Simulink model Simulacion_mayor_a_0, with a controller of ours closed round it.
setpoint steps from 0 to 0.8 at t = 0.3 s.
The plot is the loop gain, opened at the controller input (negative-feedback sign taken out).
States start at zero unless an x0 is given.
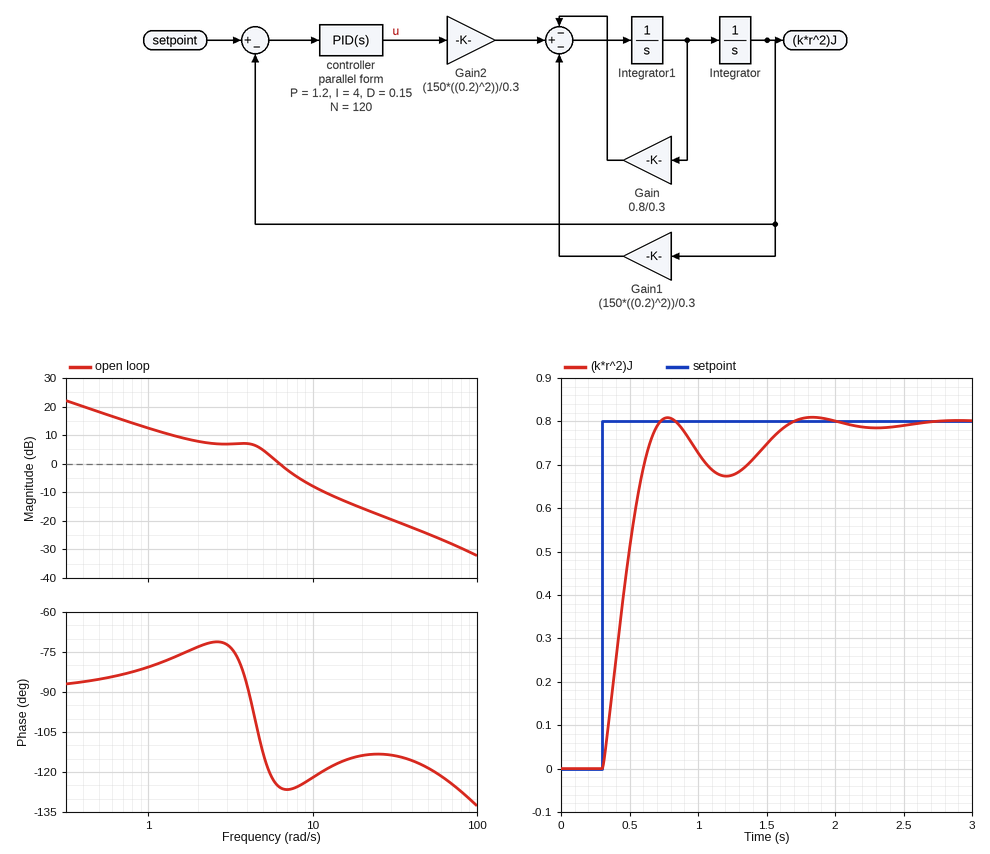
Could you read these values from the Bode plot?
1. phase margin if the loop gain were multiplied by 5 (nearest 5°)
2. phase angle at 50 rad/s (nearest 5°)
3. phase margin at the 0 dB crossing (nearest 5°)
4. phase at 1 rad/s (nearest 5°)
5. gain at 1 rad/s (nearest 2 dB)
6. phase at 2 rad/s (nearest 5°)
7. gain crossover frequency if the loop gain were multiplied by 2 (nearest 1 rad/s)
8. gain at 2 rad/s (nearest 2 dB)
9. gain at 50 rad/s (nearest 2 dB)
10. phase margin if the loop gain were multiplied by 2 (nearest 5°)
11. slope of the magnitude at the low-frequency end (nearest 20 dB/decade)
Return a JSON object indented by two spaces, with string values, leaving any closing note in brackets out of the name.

{
  "phase margin if the loop gain were multiplied by 5": "65°",
  "phase angle at 50 rad/s": "-120°",
  "phase margin at the 0 dB crossing": "55°",
  "phase at 1 rad/s": "-80°",
  "gain at 1 rad/s": "12 dB",
  "phase at 2 rad/s": "-75°",
  "gain crossover frequency if the loop gain were multiplied by 2": "9 rad/s",
  "gain at 2 rad/s": "8 dB",
  "gain at 50 rad/s": "-24 dB",
  "phase margin if the loop gain were multiplied by 2": "55°",
  "slope of the magnitude at the low-frequency end": "-20 dB/decade"
}
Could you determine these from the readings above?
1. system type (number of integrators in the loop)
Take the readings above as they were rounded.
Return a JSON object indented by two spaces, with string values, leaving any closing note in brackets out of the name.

{
  "system type": "1"
}
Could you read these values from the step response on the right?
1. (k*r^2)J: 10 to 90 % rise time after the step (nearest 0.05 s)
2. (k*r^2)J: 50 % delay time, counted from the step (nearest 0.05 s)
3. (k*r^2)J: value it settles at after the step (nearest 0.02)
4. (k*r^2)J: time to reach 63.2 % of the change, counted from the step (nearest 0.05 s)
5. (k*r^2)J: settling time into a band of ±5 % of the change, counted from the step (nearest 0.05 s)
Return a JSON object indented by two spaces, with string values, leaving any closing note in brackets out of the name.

{
  "(k*r^2)J: 10 to 90 % rise time after the step": "0.30 s",
  "(k*r^2)J: 50 % delay time, counted from the step": "0.15 s",
  "(k*r^2)J: value it settles at after the step": "0.80",
  "(k*r^2)J: time to reach 63.2 % of the change, counted from the step": "0.20 s",
  "(k*r^2)J: settling time into a band of ±5 % of the change, counted from the step": "1.25 s"
}
